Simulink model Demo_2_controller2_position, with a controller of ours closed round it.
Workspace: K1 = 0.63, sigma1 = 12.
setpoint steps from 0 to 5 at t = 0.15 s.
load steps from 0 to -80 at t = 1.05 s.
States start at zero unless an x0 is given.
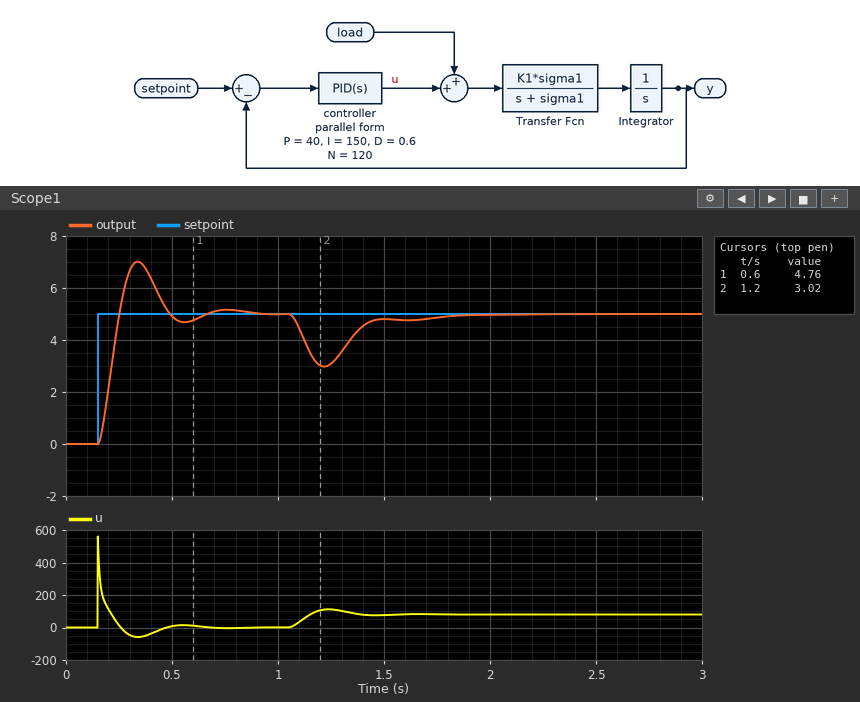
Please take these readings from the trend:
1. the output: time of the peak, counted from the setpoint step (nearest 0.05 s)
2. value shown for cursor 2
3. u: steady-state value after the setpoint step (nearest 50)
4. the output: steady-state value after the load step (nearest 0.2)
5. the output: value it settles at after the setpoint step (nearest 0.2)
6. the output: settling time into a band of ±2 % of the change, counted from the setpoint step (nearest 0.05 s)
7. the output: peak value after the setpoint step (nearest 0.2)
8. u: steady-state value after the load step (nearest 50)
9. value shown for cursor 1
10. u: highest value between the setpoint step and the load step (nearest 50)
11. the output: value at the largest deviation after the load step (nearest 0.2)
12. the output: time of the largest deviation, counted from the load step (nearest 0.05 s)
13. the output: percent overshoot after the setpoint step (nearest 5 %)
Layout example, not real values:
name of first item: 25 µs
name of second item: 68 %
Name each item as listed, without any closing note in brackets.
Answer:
the output: time of the peak, counted from the setpoint step: 0.20 s
value shown for cursor 2: 3.02
u: steady-state value after the setpoint step: 0
the output: steady-state value after the load step: 5.0
the output: value it settles at after the setpoint step: 5.0
the output: settling time into a band of ±2 % of the change, counted from the setpoint step: 0.70 s
the output: peak value after the setpoint step: 7.0
u: steady-state value after the load step: 100
value shown for cursor 1: 4.76
u: highest value between the setpoint step and the load step: 550
the output: value at the largest deviation after the load step: 3.0
the output: time of the largest deviation, counted from the load step: 0.15 s
the output: percent overshoot after the setpoint step: 40 %
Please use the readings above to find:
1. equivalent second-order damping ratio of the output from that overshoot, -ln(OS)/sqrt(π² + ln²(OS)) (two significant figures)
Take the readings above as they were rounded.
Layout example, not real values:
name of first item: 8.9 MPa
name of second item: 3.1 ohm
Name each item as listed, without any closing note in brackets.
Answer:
equivalent second-order damping ratio of the output from that overshoot, -ln(OS)/sqrt(π² + ln²(OS)): 0.28
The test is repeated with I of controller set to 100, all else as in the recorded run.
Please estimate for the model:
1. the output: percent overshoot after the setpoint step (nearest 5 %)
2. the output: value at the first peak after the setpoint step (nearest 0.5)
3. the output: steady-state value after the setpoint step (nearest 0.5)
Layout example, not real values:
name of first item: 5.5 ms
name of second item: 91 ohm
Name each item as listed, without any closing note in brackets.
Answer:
the output: percent overshoot after the setpoint step: 35 %
the output: value at the first peak after the setpoint step: 6.5
the output: steady-state value after the setpoint step: 5.0
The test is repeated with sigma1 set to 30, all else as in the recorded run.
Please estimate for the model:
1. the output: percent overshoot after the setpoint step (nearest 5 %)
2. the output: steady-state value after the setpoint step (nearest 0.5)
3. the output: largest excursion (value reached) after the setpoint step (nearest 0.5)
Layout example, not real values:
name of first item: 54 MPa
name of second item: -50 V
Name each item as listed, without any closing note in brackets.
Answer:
the output: percent overshoot after the setpoint step: 15 %
the output: steady-state value after the setpoint step: 5.0
the output: largest excursion (value reached) after the setpoint step: 6.0
